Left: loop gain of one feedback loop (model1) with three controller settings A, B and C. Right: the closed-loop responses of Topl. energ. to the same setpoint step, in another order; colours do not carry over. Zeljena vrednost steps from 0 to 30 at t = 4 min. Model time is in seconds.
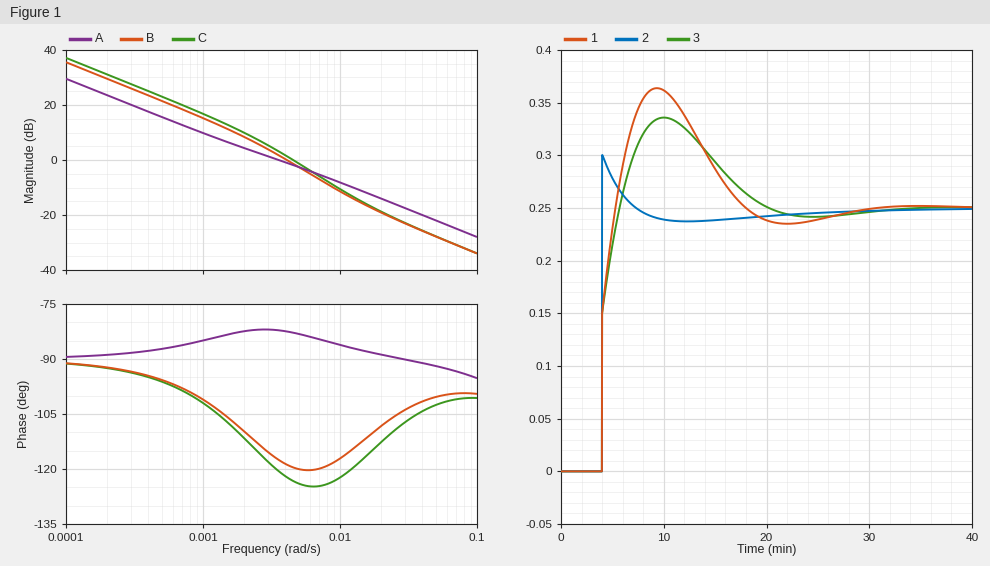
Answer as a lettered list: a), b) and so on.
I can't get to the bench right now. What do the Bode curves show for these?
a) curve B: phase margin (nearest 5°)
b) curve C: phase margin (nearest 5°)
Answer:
a) 60°
b) 55°
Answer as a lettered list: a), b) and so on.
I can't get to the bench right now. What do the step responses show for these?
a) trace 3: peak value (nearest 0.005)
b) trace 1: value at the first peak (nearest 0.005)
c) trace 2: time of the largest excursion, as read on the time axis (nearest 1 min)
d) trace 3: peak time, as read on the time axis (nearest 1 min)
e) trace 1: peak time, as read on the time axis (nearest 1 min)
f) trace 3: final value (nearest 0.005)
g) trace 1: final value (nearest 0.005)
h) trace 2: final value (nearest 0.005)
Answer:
a) 0.335
b) 0.365
c) 4 min
d) 10 min
e) 9 min
f) 0.250
g) 0.250
h) 0.250
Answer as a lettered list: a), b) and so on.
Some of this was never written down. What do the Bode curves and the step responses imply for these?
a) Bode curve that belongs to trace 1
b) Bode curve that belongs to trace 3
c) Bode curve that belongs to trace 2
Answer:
a) C
b) B
c) A
